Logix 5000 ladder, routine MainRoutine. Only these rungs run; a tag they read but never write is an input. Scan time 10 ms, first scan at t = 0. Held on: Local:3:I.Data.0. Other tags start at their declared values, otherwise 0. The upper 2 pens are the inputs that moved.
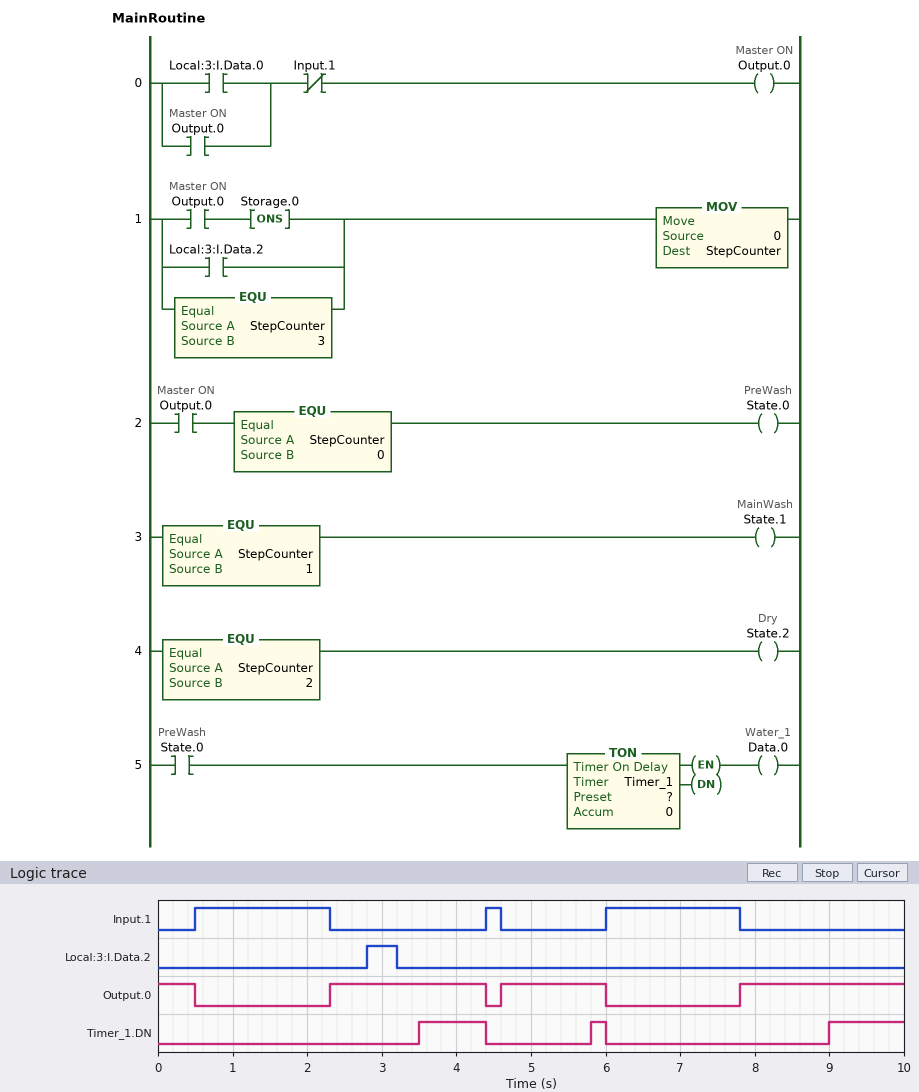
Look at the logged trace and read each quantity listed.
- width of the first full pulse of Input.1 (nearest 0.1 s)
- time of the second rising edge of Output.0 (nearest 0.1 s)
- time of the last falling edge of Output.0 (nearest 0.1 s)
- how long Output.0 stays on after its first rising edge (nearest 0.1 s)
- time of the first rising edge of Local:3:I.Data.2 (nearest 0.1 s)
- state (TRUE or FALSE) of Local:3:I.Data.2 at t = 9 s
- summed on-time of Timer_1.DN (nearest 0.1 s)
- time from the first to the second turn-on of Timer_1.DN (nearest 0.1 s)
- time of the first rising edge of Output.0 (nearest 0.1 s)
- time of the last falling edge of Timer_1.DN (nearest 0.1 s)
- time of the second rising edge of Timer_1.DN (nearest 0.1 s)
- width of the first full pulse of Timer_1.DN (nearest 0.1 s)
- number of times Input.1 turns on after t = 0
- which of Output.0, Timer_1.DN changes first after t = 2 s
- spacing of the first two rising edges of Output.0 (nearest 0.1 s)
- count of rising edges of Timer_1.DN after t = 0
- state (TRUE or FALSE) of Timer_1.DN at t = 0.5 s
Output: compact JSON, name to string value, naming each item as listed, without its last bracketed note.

{"width of the first full pulse of Input.1": "1.8 s", "time of the second rising edge of Output.0": "4.6 s", "time of the last falling edge of Output.0": "6.0 s", "how long Output.0 stays on after its first rising edge": "2.1 s", "time of the first rising edge of Local:3:I.Data.2": "2.8 s", "state (TRUE or FALSE) of Local:3:I.Data.2 at t = 9 s": "FALSE", "summed on-time of Timer_1.DN": "2.1 s", "time from the first to the second turn-on of Timer_1.DN": "2.3 s", "time of the first rising edge of Output.0": "2.3 s", "time of the last falling edge of Timer_1.DN": "6.0 s", "time of the second rising edge of Timer_1.DN": "5.8 s", "width of the first full pulse of Timer_1.DN": "0.9 s", "number of times Input.1 turns on after t = 0": "3", "which of Output.0, Timer_1.DN changes first after t = 2 s": "Output.0", "spacing of the first two rising edges of Output.0": "2.3 s", "count of rising edges of Timer_1.DN after t = 0": "3", "state (TRUE or FALSE) of Timer_1.DN at t = 0.5 s": "FALSE"}
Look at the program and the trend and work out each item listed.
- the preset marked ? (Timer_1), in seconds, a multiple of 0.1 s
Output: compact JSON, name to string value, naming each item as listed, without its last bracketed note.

{"the preset marked ? (Timer_1), in seconds, a multiple of 0.1 s": "1.2 s"}
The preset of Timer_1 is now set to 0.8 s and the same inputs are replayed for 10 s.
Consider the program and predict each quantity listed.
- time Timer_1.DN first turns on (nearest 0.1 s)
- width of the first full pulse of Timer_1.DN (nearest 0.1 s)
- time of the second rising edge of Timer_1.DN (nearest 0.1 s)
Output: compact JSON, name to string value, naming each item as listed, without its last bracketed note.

{"time Timer_1.DN first turns on": "3.1 s", "width of the first full pulse of Timer_1.DN": "1.3 s", "time of the second rising edge of Timer_1.DN": "5.4 s"}
